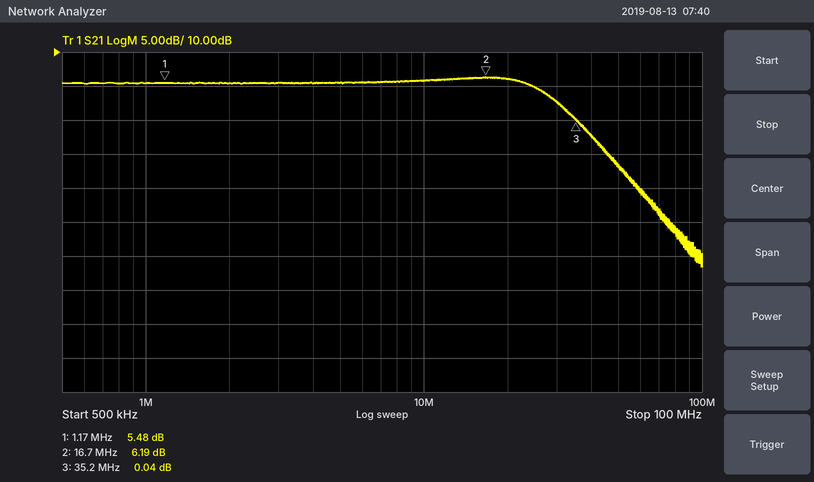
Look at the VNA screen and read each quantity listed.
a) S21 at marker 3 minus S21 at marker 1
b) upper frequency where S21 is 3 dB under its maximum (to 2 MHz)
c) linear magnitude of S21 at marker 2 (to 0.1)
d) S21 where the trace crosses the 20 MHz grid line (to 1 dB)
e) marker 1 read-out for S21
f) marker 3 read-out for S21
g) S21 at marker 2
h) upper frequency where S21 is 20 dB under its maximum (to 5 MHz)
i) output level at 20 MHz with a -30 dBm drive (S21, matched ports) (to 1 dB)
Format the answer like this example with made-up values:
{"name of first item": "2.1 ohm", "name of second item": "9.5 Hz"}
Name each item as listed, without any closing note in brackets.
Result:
{"S21 at marker 3 minus S21 at marker 1": "-5.44 dB", "upper frequency where S21 is 3 dB under its maximum": "28 MHz", "linear magnitude of S21 at marker 2": "2.0", "S21 where the trace crosses the 20 MHz grid line": "6 dB", "marker 1 read-out for S21": "5.48 dB", "marker 3 read-out for S21": "0.04 dB", "S21 at marker 2": "6.19 dB", "upper frequency where S21 is 20 dB under its maximum": "70 MHz", "output level at 20 MHz with a -30 dBm drive (S21, matched ports)": "-24 dBm"}
